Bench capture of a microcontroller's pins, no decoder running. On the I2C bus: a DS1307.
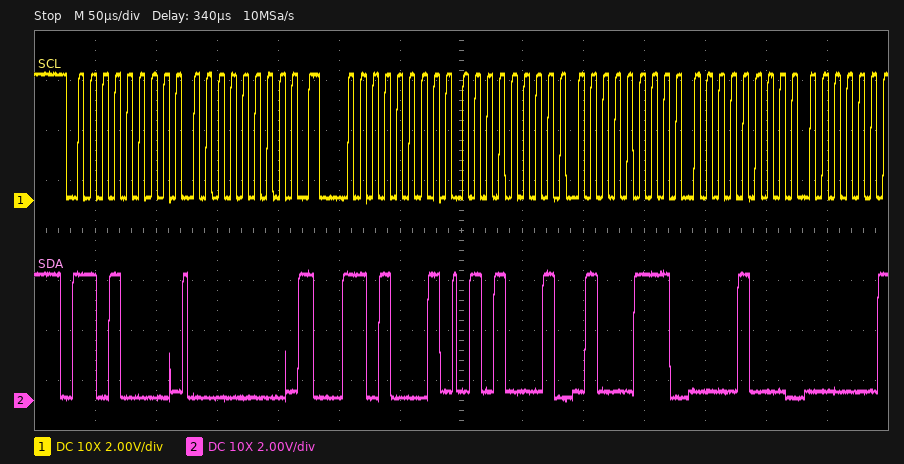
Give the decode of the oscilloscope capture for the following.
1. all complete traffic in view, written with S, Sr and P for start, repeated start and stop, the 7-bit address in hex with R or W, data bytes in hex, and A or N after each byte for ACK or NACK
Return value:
S 68W A 00 A Sr 68R A 51 A 47 A 08 A
